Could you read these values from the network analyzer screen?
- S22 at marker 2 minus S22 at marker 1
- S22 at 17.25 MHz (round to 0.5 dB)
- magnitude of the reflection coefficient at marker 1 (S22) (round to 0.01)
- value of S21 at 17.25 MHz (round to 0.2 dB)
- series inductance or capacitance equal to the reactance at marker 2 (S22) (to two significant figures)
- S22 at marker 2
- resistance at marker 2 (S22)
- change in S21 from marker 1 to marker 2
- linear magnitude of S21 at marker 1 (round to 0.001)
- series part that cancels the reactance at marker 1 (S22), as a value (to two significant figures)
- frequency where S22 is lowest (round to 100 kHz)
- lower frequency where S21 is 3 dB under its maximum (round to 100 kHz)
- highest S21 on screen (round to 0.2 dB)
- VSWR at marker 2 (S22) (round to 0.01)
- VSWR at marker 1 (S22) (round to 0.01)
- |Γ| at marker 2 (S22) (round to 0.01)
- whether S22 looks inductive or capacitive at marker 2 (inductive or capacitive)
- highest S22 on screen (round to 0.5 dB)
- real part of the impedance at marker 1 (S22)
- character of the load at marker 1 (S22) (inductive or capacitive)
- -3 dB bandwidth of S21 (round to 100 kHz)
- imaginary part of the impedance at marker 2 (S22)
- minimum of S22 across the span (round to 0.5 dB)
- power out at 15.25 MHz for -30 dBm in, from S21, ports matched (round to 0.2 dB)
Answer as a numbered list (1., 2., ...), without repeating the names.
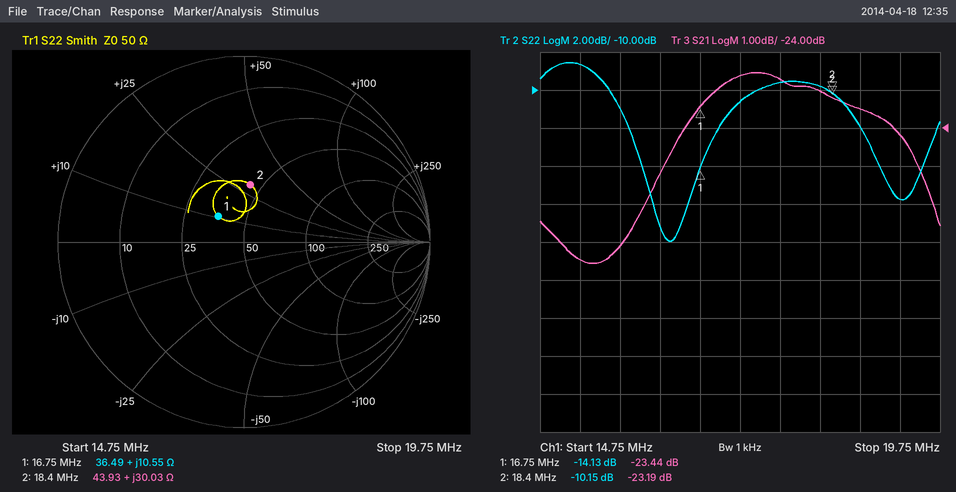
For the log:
1. 3.98 dB
2. -10.5 dB
3. 0.20
4. -22.6 dB
5. 260 nH
6. -10.15 dB
7. 43.93 Ω
8. 0.25 dB
9. 0.067
10. 900 pF
11. 16.4 MHz
12. 16.2 MHz
13. -22.6 dB
14. 1.90
15. 1.49
16. 0.31
17. inductive
18. -8.5 dB
19. 36.49 Ω
20. inductive
21. 3.4 MHz
22. +30.03 Ω
23. -18.0 dB
24. -57.4 dBm
